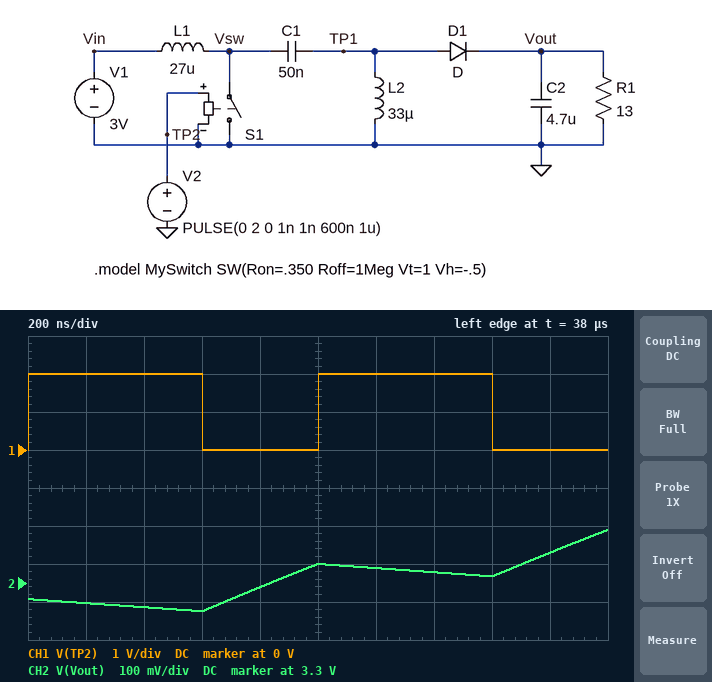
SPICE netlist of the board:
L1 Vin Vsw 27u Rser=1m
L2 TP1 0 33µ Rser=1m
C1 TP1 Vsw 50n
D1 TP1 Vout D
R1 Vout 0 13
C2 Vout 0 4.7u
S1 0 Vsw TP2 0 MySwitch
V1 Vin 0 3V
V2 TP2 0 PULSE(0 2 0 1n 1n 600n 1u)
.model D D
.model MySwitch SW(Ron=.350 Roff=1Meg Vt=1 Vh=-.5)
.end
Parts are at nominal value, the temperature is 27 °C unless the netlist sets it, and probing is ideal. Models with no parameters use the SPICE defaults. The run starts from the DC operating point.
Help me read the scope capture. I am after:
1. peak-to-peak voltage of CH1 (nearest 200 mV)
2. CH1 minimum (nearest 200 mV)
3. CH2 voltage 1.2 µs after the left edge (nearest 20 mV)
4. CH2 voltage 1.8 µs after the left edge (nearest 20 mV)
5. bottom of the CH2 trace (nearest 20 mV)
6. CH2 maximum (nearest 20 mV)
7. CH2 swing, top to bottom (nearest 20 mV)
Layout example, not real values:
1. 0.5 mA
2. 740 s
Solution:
1. 2.0 V
2. 0 V
3. 3.34 V
4. 3.38 V
5. 3.22 V
6. 3.44 V
7. 220 mV
